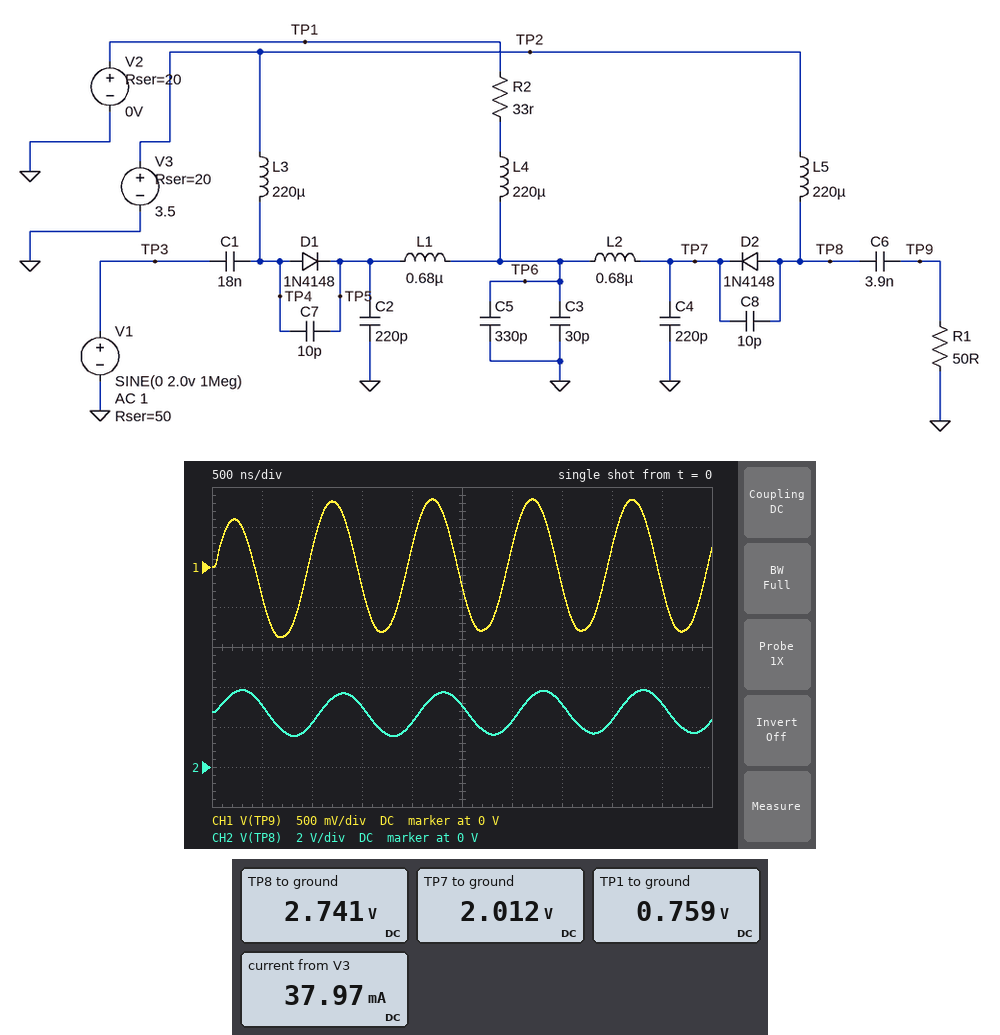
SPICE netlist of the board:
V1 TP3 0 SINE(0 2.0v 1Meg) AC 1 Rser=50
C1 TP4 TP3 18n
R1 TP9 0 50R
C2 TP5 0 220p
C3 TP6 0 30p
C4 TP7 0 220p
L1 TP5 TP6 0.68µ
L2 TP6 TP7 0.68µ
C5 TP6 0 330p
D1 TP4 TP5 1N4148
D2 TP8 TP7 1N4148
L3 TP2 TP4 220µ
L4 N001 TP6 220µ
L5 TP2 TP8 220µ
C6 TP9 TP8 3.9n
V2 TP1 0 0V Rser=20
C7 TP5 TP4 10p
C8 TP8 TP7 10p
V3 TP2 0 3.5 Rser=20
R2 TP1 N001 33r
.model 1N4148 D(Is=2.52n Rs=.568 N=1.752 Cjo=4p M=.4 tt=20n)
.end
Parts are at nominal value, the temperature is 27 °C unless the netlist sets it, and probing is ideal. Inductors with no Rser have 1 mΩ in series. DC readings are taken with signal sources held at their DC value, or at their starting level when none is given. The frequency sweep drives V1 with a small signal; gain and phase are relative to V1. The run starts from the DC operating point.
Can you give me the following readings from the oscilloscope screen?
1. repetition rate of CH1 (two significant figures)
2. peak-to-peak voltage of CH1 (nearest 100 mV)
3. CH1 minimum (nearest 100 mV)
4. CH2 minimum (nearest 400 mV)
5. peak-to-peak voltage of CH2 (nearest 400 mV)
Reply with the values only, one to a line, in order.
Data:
1.0 MHz
1.7 V
-900 mV
1.6 V
2.4 V
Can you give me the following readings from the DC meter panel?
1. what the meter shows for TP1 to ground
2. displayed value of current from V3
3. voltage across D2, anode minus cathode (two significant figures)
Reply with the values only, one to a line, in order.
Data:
0.759 V
37.97 mA
730 mV
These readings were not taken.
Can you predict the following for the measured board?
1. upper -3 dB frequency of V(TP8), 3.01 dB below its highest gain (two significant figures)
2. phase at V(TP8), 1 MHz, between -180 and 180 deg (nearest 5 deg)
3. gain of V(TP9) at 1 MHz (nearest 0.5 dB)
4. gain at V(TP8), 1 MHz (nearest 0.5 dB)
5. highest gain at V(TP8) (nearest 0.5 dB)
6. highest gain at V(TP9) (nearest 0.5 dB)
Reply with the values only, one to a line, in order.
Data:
400 kHz
-20 deg
-7.5 dB
-5.0 dB
0.5 dB
-6.0 dB
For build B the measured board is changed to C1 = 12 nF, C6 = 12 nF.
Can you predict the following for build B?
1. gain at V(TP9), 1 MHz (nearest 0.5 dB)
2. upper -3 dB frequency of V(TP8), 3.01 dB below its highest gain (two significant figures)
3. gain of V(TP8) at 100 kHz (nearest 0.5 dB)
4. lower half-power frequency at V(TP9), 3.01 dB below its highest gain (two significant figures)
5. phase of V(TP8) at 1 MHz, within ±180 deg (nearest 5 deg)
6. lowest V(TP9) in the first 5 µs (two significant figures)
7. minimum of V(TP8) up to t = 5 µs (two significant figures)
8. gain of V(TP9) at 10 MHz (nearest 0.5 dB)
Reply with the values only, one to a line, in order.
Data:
-7.0 dB
320 kHz
-5.5 dB
140 kHz
-10 deg
-960 mV
1.8 V
-6.5 dB
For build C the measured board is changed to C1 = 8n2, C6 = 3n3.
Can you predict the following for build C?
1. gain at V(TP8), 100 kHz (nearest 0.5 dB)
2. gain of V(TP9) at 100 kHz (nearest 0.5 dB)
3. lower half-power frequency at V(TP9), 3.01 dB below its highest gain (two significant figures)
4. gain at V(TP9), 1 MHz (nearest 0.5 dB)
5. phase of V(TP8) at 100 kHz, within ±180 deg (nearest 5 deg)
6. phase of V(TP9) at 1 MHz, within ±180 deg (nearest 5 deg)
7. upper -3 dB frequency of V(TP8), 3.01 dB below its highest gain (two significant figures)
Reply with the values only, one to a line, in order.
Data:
-9.5 dB
-29.0 dB
660 kHz
-8.0 dB
135 deg
25 deg
280 kHz
